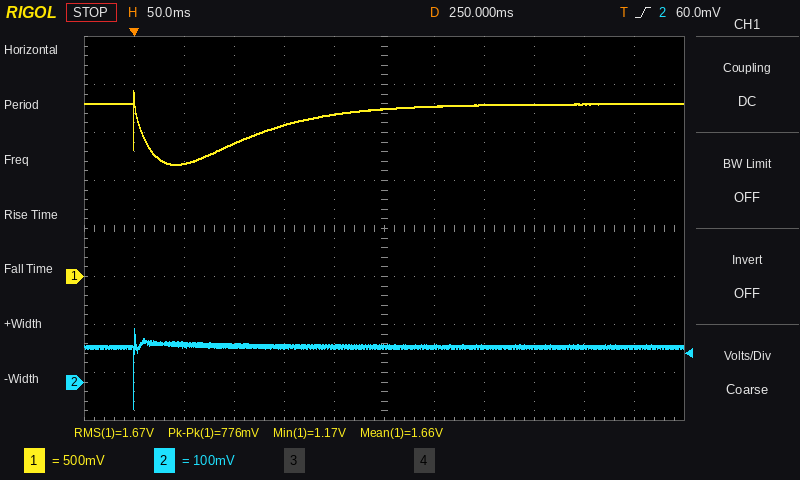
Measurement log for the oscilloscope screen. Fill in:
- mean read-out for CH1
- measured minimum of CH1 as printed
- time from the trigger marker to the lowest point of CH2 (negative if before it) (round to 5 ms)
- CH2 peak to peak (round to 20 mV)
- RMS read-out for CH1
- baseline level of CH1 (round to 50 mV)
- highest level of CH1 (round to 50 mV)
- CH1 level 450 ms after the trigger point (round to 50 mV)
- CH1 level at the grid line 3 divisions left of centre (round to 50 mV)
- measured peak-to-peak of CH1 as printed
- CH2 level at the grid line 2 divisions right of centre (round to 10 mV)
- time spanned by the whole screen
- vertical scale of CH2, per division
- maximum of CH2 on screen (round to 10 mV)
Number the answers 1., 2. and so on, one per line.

1. 1.66 V
2. 1.17 V
3. 0 ms
4. 160 mV
5. 1.67 V
6. 1.80 V
7. 1.95 V
8. 1.80 V
9. 1.40 V
10. 776 mV
11. 70 mV
12. 600 ms
13. 100 mV
14. 110 mV
